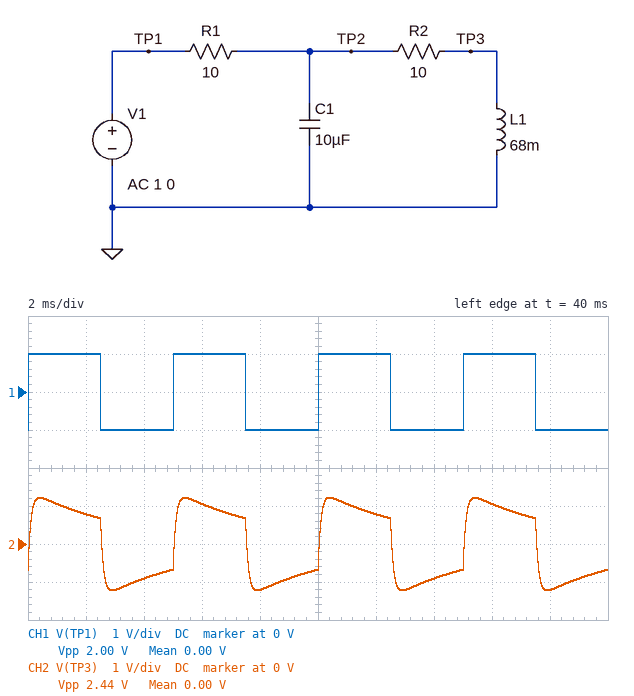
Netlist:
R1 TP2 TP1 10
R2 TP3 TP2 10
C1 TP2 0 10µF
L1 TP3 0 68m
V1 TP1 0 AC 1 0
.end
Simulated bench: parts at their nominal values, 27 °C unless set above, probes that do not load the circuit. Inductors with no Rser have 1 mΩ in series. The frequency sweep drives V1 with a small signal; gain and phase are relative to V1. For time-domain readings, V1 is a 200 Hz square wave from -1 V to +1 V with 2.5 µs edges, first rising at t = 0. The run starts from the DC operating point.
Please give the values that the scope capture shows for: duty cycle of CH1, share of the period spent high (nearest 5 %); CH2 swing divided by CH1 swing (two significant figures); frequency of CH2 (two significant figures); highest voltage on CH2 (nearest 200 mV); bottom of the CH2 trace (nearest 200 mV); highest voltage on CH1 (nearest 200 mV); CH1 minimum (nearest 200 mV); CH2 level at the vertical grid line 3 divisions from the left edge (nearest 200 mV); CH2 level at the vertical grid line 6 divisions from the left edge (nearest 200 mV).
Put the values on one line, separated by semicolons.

50 %; 1.2; 200 Hz; 1.2 V; -1.2 V; 1.0 V; -1.0 V; 1.0 V; 800 mV
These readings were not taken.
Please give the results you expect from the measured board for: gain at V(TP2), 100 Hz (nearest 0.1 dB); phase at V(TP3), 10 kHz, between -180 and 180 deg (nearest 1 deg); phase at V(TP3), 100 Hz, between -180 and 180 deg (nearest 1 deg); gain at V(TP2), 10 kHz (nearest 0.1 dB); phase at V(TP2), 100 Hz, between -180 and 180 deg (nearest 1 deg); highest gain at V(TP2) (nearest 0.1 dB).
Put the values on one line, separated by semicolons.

-0.5 dB; -81 deg; 22 deg; -16.1 dB; 9 deg; -0.1 dB
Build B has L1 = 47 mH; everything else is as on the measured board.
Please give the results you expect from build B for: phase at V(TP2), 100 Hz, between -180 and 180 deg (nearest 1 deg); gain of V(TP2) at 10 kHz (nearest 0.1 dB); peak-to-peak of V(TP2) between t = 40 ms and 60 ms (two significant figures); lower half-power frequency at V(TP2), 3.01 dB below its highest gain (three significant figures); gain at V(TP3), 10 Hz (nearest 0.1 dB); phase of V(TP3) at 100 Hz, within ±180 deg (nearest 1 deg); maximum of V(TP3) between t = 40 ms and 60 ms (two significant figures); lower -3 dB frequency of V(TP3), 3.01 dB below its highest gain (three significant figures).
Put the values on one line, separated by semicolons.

12 deg; -16.1 dB; 2.3 V; 44.9 Hz; -16.7 dB; 31 deg; 1.3 V; 63.8 Hz
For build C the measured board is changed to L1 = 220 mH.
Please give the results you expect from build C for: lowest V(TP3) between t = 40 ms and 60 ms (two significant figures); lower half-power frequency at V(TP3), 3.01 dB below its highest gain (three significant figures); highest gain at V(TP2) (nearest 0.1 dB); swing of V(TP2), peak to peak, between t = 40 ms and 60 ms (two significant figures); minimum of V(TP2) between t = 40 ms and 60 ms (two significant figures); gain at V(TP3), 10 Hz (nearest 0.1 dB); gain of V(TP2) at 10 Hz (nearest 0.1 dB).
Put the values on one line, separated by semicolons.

-1.1 V; 14.3 Hz; 0 dB; 2.1 V; -1.0 V; -4.9 dB; -3.1 dB
